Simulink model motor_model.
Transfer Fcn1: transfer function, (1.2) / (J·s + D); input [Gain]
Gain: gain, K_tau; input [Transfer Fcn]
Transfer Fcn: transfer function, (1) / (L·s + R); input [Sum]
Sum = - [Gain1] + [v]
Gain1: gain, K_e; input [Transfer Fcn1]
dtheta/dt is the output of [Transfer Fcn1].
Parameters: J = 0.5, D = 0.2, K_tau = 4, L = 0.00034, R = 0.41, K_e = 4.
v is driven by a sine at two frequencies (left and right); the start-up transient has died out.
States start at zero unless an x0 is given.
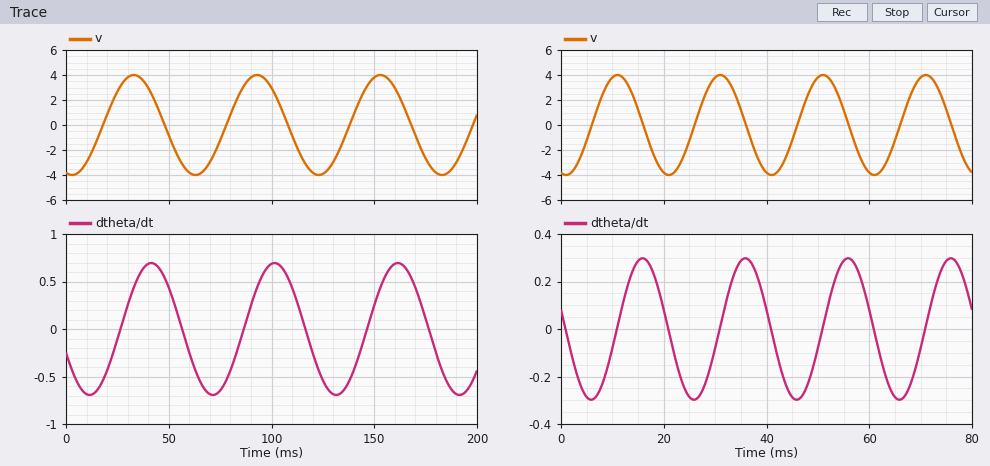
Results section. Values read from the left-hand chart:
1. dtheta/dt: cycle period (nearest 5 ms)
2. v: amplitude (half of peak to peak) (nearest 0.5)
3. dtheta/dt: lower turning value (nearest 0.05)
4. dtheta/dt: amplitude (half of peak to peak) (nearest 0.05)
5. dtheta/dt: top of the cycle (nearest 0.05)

60 ms
4.0
-0.70
0.70
0.70
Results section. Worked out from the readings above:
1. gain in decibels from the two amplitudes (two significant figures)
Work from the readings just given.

-15 dB
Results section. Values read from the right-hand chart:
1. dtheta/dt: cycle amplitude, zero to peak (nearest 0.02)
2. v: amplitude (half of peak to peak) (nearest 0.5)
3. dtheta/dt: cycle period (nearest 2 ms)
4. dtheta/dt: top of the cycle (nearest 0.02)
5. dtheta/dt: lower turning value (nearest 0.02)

0.30
4.0
20 ms
0.30
-0.30
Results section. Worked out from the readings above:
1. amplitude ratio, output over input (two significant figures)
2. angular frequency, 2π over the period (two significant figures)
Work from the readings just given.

0.075
0.31 rad/ms
